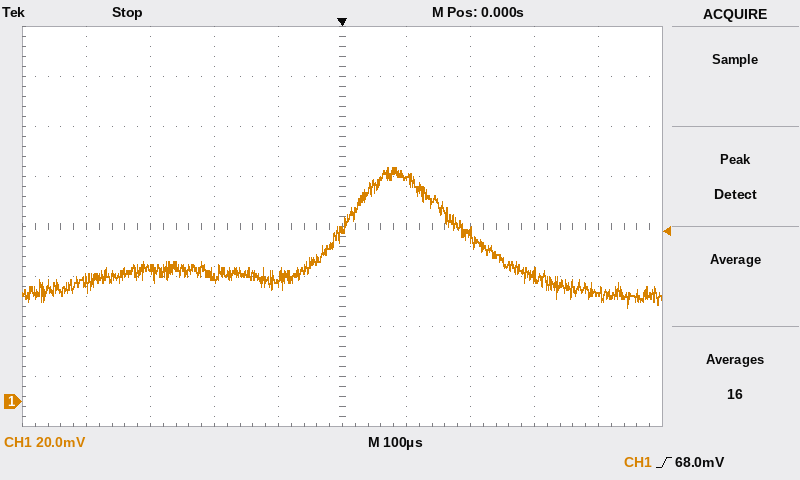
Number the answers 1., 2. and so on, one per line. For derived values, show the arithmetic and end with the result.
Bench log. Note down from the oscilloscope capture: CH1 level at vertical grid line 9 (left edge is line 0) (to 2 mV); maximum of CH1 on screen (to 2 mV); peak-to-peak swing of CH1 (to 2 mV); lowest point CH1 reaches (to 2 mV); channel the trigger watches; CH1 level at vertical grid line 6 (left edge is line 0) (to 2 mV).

1. 44 mV
2. 94 mV
3. 94 mV − (38 mV) = 56 mV
4. 38 mV
5. CH1
6. 90 mV
